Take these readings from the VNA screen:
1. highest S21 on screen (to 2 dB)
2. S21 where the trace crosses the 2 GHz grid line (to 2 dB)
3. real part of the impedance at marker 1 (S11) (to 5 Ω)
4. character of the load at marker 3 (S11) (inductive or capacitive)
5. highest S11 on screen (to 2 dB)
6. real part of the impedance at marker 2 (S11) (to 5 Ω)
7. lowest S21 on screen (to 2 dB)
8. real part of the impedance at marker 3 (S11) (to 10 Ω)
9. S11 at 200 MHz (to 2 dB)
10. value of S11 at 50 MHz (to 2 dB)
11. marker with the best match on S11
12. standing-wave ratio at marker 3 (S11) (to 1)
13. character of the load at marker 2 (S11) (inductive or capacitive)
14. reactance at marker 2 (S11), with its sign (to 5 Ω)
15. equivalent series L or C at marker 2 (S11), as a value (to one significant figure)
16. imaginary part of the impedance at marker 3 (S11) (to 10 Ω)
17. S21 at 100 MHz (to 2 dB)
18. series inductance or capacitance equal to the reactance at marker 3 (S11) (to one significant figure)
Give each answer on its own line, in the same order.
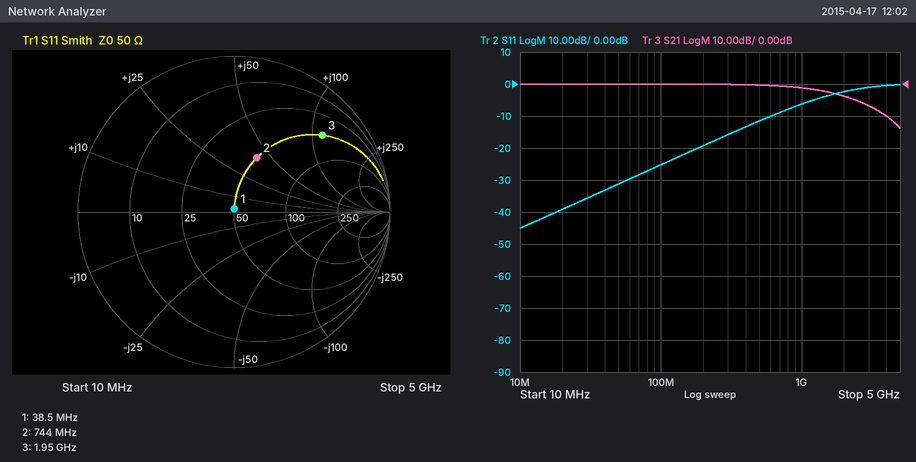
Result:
0 dB
-4 dB
50 Ω
inductive
0 dB
50 Ω
-14 dB
50 Ω
-20 dB
-32 dB
marker 1
7
inductive
+40 Ω
9 nH
+110 Ω
0 dB
9 nH
